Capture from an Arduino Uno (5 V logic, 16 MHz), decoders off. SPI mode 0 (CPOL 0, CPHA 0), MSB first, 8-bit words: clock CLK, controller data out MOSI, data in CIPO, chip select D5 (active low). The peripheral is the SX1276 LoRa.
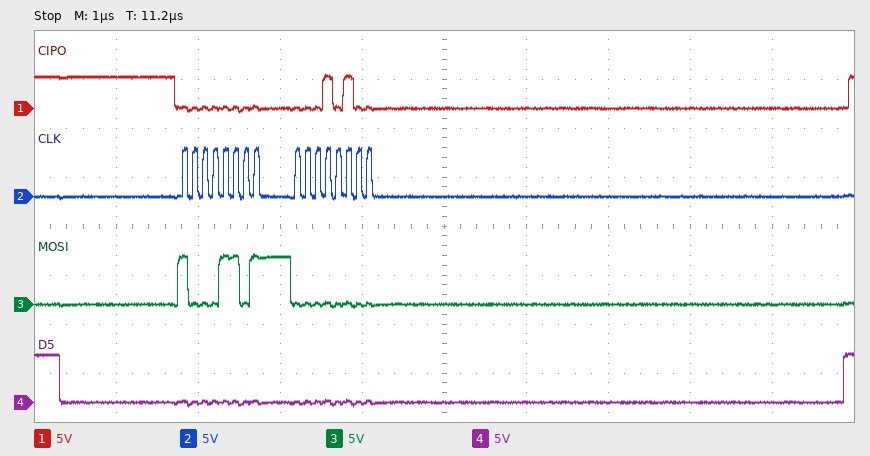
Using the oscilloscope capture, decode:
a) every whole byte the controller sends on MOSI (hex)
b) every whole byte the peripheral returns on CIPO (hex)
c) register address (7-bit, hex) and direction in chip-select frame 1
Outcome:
0x8D 0x00
0x00 0x14
0x0D write
